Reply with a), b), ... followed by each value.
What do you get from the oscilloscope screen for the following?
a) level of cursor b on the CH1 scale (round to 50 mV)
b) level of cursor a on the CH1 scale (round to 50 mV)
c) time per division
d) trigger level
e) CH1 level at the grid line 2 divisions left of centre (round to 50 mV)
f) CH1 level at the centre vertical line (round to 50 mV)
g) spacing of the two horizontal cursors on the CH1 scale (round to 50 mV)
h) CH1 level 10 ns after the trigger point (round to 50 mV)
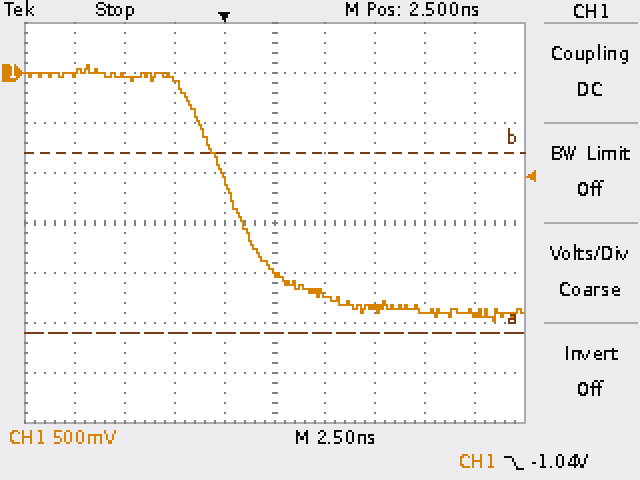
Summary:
a) -800 mV
b) -2.60 V
c) 2.5 ns
d) -1.04 V
e) -50 mV
f) -2.00 V
g) 1.80 V
h) -2.40 V
